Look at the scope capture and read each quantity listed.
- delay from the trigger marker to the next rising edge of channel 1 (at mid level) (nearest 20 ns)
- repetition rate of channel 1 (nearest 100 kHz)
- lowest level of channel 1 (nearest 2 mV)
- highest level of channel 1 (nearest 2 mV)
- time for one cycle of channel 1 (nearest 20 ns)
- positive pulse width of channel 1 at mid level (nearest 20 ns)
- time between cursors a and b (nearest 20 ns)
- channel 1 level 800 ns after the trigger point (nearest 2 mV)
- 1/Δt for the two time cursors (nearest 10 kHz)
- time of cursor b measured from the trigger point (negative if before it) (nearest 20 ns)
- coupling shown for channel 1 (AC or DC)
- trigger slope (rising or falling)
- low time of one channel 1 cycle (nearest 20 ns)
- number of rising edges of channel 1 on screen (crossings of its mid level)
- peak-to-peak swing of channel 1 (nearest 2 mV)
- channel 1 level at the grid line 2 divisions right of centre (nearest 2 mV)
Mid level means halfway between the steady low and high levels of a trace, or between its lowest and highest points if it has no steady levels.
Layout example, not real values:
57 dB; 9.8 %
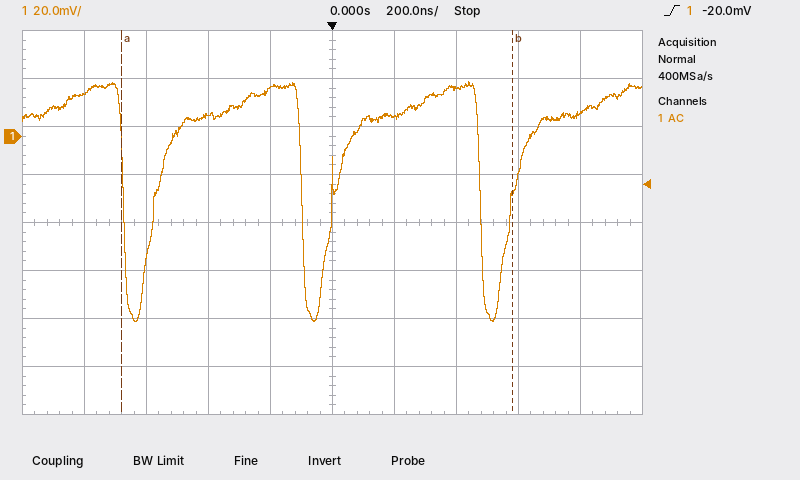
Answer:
580 ns; 1.7 MHz; -78 mV; 22 mV; 580 ns; 480 ns; 1.26 µs; 10 mV; 790 kHz; +580 ns; AC; rising; 100 ns; 3; 100 mV; 20 mV
